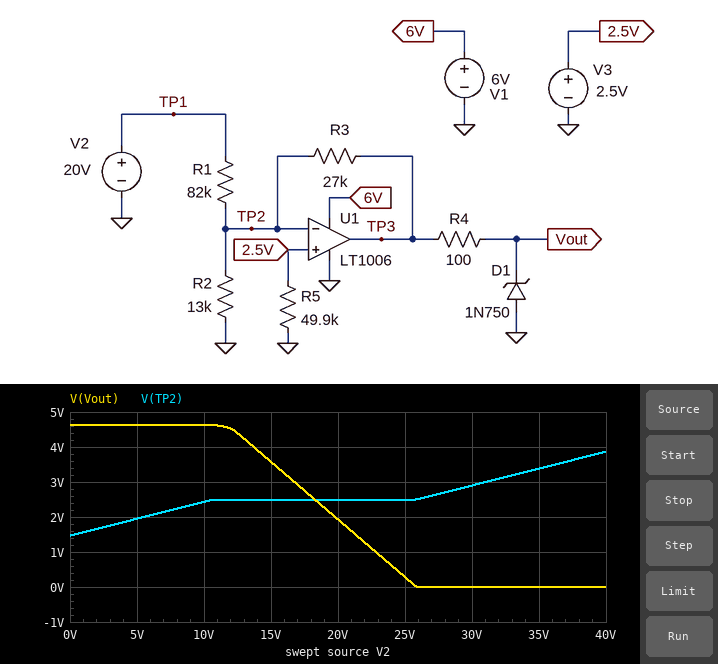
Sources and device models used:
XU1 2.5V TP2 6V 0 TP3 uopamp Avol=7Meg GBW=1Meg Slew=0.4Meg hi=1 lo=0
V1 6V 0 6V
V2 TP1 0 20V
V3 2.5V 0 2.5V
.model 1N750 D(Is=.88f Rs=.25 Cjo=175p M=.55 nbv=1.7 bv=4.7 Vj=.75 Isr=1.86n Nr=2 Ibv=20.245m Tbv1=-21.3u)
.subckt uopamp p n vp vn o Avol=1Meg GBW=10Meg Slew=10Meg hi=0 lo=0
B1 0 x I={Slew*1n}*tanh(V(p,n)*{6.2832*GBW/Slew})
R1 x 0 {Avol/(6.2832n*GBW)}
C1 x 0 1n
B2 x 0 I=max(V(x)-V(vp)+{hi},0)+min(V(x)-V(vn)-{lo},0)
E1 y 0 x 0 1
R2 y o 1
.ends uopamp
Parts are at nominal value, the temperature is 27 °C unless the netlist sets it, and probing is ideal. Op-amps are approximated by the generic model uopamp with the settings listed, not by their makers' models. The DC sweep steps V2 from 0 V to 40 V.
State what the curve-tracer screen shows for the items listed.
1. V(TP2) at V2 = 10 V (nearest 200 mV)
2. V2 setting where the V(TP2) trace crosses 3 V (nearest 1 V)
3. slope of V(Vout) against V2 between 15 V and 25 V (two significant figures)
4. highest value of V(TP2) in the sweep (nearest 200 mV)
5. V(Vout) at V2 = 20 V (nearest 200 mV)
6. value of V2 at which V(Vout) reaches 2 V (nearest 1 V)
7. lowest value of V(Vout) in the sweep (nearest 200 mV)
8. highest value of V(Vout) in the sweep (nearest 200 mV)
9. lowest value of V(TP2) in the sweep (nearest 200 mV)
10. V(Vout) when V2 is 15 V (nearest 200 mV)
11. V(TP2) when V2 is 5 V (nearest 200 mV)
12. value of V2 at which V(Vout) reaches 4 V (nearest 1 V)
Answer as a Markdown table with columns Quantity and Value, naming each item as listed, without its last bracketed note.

| Quantity | Value |
|---|---|
| V(TP2) at V2 = 10 V | 2.4 V |
| V2 setting where the V(TP2) trace crosses 3 V | 31 V |
| slope of V(Vout) against V2 between 15 V and 25 V | -0.33 V/V |
| highest value of V(TP2) in the sweep | 3.8 V |
| V(Vout) at V2 = 20 V | 2.0 V |
| value of V2 at which V(Vout) reaches 2 V | 20 V |
| lowest value of V(Vout) in the sweep | 0 V |
| highest value of V(Vout) in the sweep | 4.6 V |
| lowest value of V(TP2) in the sweep | 1.4 V |
| V(Vout) when V2 is 15 V | 3.6 V |
| V(TP2) when V2 is 5 V | 2.0 V |
| value of V2 at which V(Vout) reaches 4 V | 14 V |
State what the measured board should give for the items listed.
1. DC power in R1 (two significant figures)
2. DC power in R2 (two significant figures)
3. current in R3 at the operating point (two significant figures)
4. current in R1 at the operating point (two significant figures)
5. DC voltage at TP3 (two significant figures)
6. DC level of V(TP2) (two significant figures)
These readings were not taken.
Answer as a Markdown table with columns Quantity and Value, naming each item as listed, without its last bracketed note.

| Quantity | Value |
|---|---|
| DC power in R1 | 3.7 mW |
| DC power in R2 | 480 µW |
| current in R3 at the operating point | 21 µA |
| current in R1 at the operating point | 210 µA |
| DC voltage at TP3 | 1.9 V |
| DC level of V(TP2) | 2.5 V |
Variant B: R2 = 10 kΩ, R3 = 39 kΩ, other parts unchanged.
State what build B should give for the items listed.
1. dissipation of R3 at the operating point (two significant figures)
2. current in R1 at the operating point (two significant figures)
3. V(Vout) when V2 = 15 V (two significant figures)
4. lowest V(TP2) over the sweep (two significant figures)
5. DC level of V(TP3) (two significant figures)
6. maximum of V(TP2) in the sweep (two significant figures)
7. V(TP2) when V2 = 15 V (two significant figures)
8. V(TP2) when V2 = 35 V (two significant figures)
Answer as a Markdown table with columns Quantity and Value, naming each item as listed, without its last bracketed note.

| Quantity | Value |
|---|---|
| dissipation of R3 at the operating point | 52 µW |
| current in R1 at the operating point | 210 µA |
| V(Vout) when V2 = 15 V | 4.6 V |
| lowest V(TP2) over the sweep | 930 mV |
| DC level of V(TP3) | 3.9 V |
| maximum of V(TP2) in the sweep | 3.5 V |
| V(TP2) when V2 = 15 V | 2.3 V |
| V(TP2) when V2 = 35 V | 3.1 V |
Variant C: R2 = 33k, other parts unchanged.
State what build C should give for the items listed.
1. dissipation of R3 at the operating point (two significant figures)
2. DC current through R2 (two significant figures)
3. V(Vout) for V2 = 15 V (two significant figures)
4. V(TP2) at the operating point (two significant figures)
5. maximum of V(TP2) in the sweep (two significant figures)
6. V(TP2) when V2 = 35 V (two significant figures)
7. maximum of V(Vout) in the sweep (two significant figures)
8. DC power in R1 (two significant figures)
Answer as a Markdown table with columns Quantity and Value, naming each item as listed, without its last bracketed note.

| Quantity | Value |
|---|---|
| dissipation of R3 at the operating point | 350 µW |
| DC current through R2 | 93 µA |
| V(Vout) for V2 = 15 V | 430 mV |
| V(TP2) at the operating point | 3.1 V |
| maximum of V(TP2) in the sweep | 6.1 V |
| V(TP2) when V2 = 35 V | 5.4 V |
| maximum of V(Vout) in the sweep | 4.6 V |
| DC power in R1 | 3.5 mW |
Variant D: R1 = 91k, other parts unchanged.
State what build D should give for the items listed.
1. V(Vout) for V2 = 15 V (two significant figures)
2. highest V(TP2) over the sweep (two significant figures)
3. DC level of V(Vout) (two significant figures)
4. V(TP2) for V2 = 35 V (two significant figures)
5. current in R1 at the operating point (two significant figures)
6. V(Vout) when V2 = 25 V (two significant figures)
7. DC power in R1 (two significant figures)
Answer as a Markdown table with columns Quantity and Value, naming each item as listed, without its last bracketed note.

| Quantity | Value |
|---|---|
| V(Vout) for V2 = 15 V | 4.0 V |
| highest V(TP2) over the sweep | 3.5 V |
| DC level of V(Vout) | 2.5 V |
| V(TP2) for V2 = 35 V | 3.1 V |
| current in R1 at the operating point | 190 µA |
| V(Vout) when V2 = 25 V | 1.0 V |
| DC power in R1 | 3.4 mW |
